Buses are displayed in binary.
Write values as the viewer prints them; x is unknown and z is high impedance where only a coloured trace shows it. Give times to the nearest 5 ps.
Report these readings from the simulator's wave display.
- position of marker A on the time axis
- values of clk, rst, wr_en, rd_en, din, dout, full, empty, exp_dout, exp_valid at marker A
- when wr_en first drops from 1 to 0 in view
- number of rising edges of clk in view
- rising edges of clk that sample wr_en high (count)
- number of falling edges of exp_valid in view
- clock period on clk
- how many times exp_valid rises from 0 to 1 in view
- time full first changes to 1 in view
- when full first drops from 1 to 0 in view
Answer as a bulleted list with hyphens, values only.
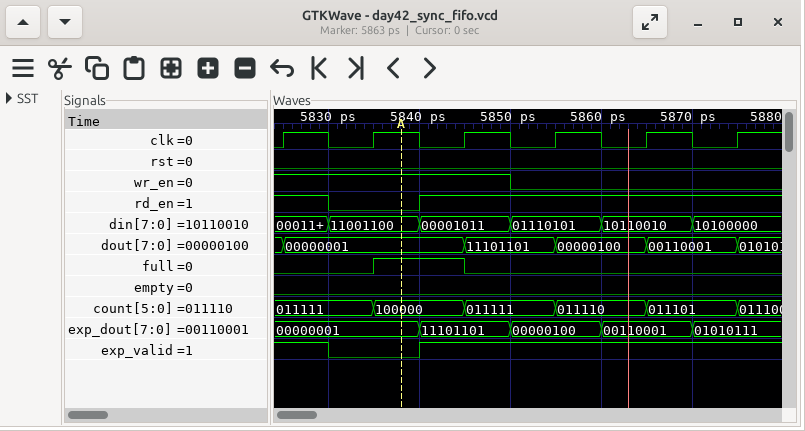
- 5840 ps
- clk=1, rst=0, wr_en=1, rd_en=0, din=11001100, dout=00000001, full=1, empty=0, exp_dout=00000001, exp_valid=0
- 5850 ps
- 6
- 3
- 1
- 10 ps
- 1
- 5835 ps
- 5845 ps
